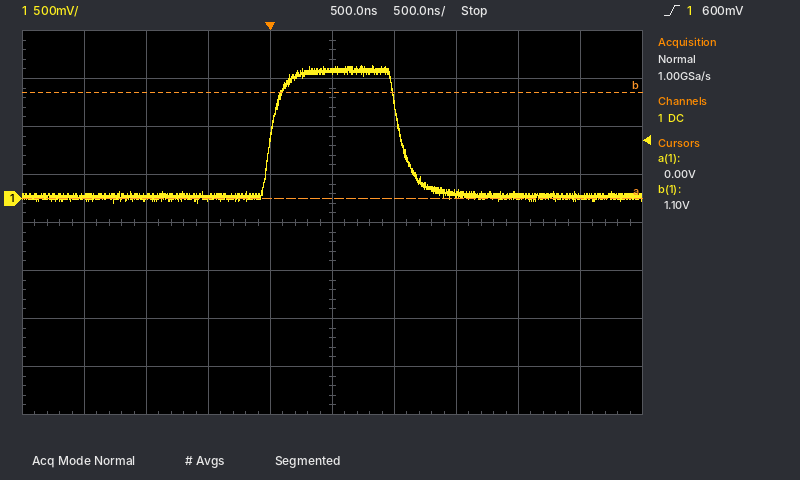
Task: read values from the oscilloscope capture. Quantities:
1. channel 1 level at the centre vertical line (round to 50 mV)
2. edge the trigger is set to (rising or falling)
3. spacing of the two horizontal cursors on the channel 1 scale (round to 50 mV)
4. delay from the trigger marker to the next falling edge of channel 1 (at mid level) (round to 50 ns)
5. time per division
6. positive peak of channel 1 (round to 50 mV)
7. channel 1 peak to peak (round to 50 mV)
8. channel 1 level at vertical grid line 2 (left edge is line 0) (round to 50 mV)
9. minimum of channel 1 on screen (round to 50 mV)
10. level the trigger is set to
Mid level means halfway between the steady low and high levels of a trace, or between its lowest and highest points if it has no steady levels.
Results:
1.30 V
rising
1.10 V
1.05 µs
500 ns
1.40 V
1.45 V
0 mV
-50 mV
600 mV
